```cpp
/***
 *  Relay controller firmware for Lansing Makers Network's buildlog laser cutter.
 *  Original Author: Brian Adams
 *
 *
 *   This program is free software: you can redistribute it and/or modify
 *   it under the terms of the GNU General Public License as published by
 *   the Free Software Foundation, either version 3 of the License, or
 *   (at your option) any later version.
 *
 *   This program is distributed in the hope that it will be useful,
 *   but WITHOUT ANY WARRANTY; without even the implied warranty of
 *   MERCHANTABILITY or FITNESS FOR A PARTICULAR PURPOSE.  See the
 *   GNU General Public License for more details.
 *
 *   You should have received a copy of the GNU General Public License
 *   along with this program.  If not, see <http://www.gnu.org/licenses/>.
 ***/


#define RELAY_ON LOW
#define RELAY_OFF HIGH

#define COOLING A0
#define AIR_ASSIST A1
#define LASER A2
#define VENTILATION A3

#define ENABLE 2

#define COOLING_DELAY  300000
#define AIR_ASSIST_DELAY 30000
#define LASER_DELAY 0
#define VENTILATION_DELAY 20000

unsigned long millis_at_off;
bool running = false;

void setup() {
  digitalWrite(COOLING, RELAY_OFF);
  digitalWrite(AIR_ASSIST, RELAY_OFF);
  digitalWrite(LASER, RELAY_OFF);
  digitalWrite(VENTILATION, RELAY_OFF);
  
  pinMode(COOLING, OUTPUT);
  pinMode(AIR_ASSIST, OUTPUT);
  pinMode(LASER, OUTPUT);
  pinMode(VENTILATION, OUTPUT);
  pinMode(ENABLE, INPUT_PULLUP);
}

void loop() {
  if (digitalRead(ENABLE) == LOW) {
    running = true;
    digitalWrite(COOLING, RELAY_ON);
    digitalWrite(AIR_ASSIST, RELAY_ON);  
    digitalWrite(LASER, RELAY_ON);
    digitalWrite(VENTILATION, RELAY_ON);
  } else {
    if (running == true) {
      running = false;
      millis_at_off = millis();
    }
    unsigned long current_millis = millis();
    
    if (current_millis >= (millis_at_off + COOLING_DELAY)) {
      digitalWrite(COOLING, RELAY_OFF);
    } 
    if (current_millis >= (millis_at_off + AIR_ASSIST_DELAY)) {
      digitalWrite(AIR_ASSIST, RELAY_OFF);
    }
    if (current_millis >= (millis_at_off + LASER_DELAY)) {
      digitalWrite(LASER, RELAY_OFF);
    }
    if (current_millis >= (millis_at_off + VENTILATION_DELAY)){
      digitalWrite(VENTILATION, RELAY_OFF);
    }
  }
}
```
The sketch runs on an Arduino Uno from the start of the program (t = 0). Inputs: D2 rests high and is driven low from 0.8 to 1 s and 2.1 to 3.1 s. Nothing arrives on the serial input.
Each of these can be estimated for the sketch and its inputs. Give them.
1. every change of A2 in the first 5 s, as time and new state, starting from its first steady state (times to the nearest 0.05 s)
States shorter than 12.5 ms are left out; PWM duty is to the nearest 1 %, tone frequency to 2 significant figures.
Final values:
0 s high; 0.8 s low; 1 s high; 2.1 s low; 3.1 s high
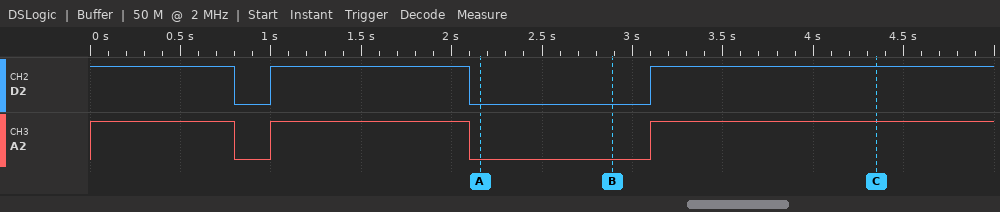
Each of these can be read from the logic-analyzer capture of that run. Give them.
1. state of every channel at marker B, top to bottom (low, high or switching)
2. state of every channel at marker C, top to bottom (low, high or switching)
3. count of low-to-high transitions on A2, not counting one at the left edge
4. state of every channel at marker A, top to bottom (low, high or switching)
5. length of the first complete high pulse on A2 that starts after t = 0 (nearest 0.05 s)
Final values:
D2 low, A2 low
D2 high, A2 high
2
D2 low, A2 low
1.10 s
